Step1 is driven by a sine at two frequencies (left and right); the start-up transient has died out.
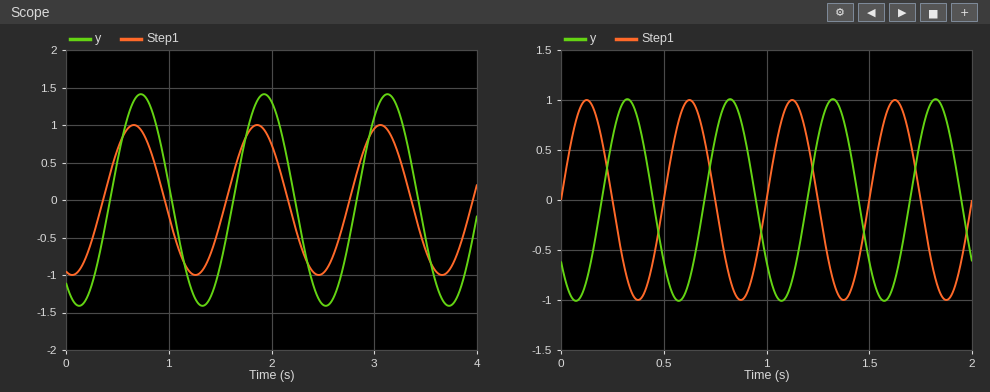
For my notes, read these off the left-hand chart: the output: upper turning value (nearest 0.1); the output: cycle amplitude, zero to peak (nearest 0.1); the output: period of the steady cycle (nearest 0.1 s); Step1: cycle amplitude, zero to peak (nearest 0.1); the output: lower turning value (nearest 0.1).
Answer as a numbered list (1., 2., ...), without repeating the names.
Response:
1. 1.4
2. 1.4
3. 1.2 s
4. 1.0
5. -1.4
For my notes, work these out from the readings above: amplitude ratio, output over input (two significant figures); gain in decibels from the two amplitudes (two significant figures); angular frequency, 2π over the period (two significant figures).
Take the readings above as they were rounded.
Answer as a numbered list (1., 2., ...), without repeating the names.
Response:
1. 1.4
2. 2.9 dB
3. 5.2 rad/s
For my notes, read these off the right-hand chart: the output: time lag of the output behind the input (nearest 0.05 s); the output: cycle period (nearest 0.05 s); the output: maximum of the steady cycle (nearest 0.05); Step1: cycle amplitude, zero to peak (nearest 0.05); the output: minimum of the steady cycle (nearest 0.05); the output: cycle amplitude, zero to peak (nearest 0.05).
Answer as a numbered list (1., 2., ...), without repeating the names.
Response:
1. 0.20 s
2. 0.50 s
3. 1.00
4. 1.00
5. -1.00
6. 1.00
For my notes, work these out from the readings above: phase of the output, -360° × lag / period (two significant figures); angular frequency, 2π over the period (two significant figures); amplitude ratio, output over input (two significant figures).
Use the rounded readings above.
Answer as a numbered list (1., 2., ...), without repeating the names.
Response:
1. -140°
2. 13 rad/s
3. 1.0
